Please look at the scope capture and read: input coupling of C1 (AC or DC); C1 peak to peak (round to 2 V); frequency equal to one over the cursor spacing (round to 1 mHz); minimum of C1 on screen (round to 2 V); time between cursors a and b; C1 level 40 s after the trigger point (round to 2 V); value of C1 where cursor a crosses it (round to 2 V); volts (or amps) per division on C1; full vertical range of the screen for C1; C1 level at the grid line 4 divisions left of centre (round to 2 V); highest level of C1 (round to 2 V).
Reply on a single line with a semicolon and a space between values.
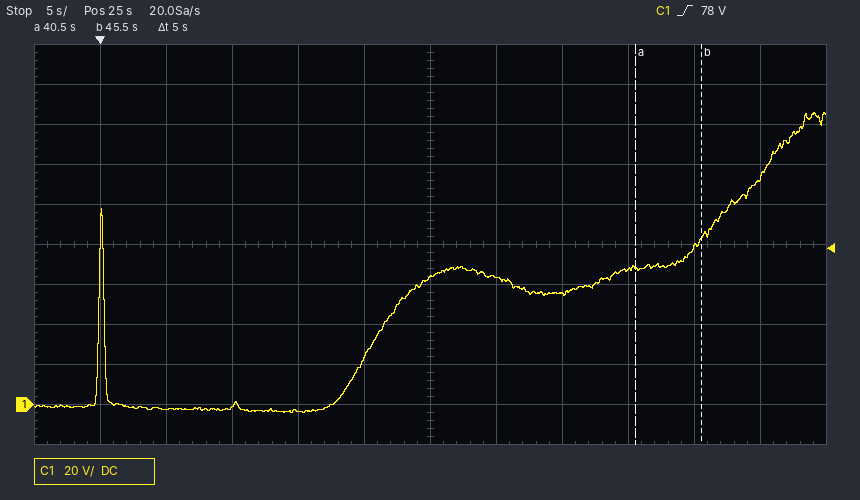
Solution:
DC; 150 V; 200 mHz; -4 V; 5 s; 68 V; 68 V; 20 V; 200 V; -2 V; 146 V
